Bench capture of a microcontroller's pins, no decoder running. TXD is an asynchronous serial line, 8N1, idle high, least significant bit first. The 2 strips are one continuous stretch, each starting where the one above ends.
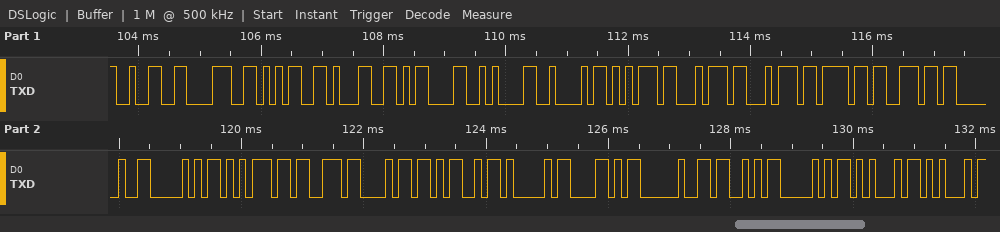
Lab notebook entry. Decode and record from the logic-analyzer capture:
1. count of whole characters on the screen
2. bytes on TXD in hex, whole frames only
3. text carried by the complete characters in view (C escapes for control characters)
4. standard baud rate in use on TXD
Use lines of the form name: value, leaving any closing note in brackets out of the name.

count of whole characters on the screen: 25
bytes on TXD in hex, whole frames only: 32 38 35 31 0D 0A 42 75 74 74 6F 6E 20 50 75 73 68 4D 41 58 20 53 50 45 45
text carried by the complete characters in view: "2851\r\nButton PushMAX SPEE"
standard baud rate in use on TXD: 9600 baud
